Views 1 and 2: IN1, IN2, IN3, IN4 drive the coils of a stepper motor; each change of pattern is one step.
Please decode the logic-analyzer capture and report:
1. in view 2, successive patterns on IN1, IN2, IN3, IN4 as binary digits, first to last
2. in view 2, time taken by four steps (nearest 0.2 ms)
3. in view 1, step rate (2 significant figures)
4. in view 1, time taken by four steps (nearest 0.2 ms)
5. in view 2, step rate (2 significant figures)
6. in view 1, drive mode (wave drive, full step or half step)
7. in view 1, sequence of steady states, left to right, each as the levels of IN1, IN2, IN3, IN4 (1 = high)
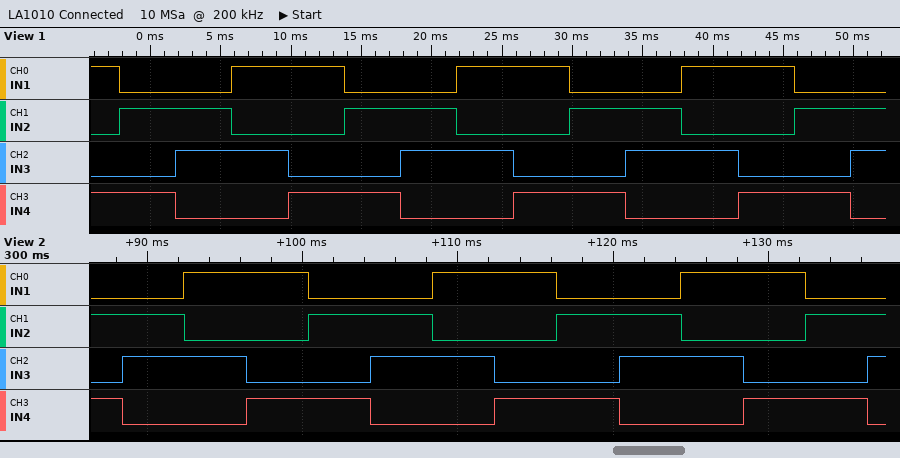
0101 0110 1010 1001 0101 0110 1010 1001 0101 0110 1010 1001 0101 0110
16.0 ms
250 steps/s
16.0 ms
250 steps/s
full step
1001 0101 0110 1010 1001 0101 0110 1010 1001 0101 0110 1010 1001 0101 0110
